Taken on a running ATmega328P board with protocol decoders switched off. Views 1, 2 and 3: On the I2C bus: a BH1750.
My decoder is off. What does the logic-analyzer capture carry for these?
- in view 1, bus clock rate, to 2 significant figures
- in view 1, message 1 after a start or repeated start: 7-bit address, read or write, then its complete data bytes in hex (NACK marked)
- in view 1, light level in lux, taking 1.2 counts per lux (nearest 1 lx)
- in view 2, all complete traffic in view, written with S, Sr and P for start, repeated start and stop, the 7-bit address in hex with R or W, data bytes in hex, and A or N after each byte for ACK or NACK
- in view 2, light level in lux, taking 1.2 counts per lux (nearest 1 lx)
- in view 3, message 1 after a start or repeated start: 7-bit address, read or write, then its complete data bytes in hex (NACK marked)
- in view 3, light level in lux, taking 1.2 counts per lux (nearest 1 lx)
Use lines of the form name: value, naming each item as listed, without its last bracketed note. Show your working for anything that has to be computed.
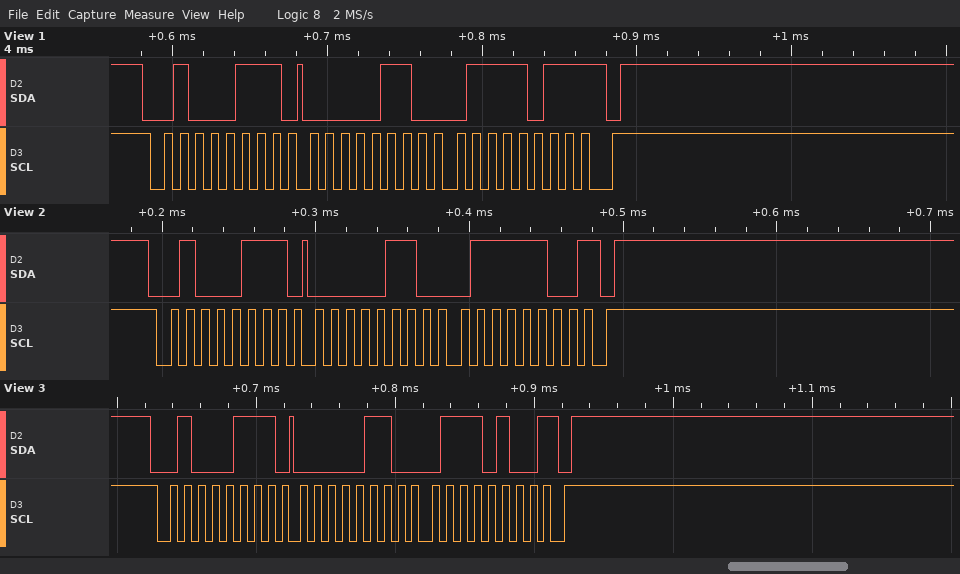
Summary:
in view 1, bus clock rate, to 2 significant figures: 100 kHz
in view 1, message 1 after a start or repeated start: 7-bit address, read or write, then its complete data bytes in hex: 0x23 read: 06 7B NACK
in view 1, light level in lux, taking 1.2 counts per lux: 1659 / 1.2 = 1382 lx
in view 2, all complete traffic in view, written with S, Sr and P for start, repeated start and stop, the 7-bit address in hex with R or W, data bytes in hex, and A or N after each byte for ACK or NACK: S 23R A 06 A 7C N P
in view 2, light level in lux, taking 1.2 counts per lux: 1660 / 1.2 = 1383 lx
in view 3, message 1 after a start or repeated start: 7-bit address, read or write, then its complete data bytes in hex: 0x23 read: 06 74 NACK
in view 3, light level in lux, taking 1.2 counts per lux: 1652 / 1.2 = 1377 lx
